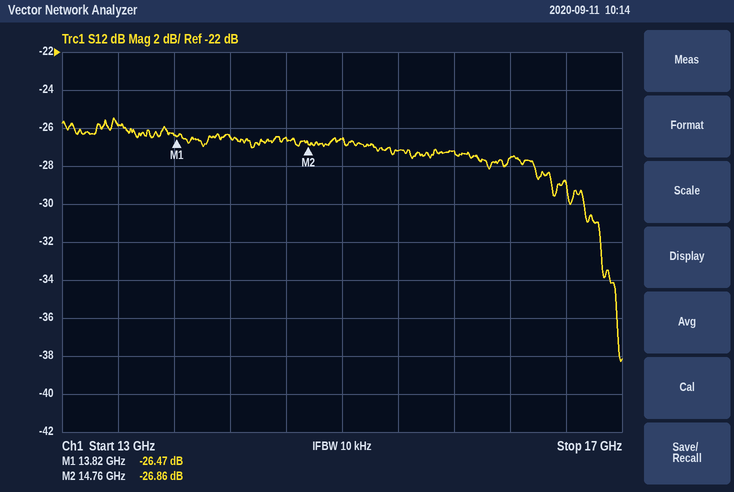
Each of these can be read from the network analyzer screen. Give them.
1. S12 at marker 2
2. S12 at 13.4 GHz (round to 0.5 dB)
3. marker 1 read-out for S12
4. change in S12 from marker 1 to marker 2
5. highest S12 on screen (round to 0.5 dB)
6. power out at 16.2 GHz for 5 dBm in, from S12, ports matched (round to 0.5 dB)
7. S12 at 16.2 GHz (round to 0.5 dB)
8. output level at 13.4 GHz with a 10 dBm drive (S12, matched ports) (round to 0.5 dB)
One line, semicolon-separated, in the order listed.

-26.86 dB; -26.0 dB; -26.47 dB; -0.39 dB; -25.5 dB; -22.5 dBm; -27.5 dB; -16.0 dBm
